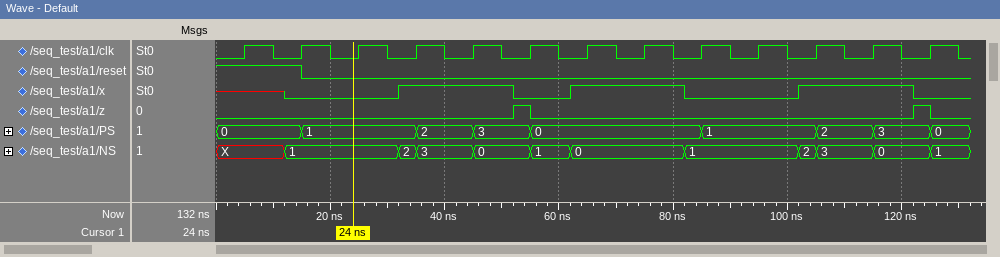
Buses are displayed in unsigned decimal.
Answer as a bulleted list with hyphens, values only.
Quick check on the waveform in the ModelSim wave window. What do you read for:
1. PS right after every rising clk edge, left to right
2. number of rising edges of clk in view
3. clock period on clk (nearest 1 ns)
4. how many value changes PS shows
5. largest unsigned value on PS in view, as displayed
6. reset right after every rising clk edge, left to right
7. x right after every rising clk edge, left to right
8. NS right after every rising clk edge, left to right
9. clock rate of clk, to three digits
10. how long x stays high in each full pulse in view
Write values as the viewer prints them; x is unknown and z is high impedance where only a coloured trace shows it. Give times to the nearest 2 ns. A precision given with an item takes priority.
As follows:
- 0, 1, 1, 2, 3, 0, 0, 0, 1, 1, 2, 3, 0
- 13
- 10 ns
- 8
- 3
- 1 0 0 0 0 0 0 0 0 0 0 0 0
- x 0 0 1 1 0 1 1 0 0 1 1 0
- X, 1, 1, 3, 0, 1, 0, 0, 1, 1, 3, 0, 1
- 100 MHz
- 20 ns, 20 ns, 20 ns
